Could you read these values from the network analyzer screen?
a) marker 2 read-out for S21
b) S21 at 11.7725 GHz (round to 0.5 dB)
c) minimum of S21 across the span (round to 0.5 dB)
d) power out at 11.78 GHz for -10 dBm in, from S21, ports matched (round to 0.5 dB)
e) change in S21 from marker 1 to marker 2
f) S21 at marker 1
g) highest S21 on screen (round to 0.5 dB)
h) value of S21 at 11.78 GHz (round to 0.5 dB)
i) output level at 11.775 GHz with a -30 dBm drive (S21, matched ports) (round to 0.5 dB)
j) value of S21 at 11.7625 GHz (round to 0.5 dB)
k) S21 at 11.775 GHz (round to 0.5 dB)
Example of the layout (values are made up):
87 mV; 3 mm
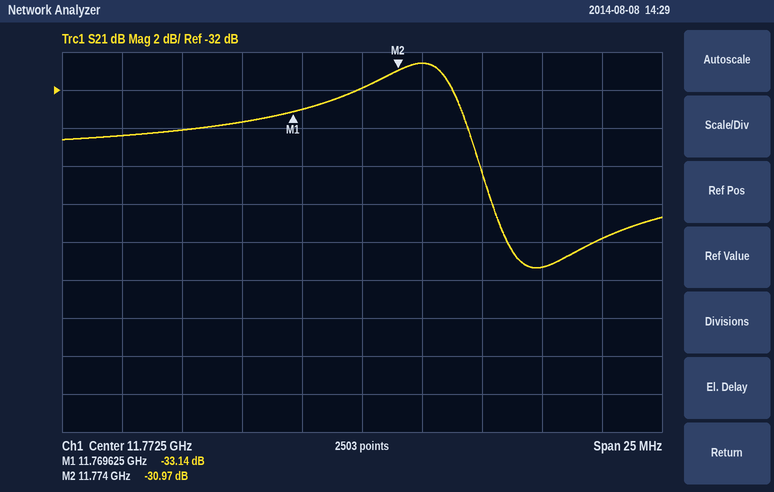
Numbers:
-30.97 dB; -32.0 dB; -41.5 dB; -51.5 dBm; 2.17 dB; -33.14 dB; -30.5 dB; -41.5 dB; -60.5 dBm; -34.5 dB; -30.5 dB
